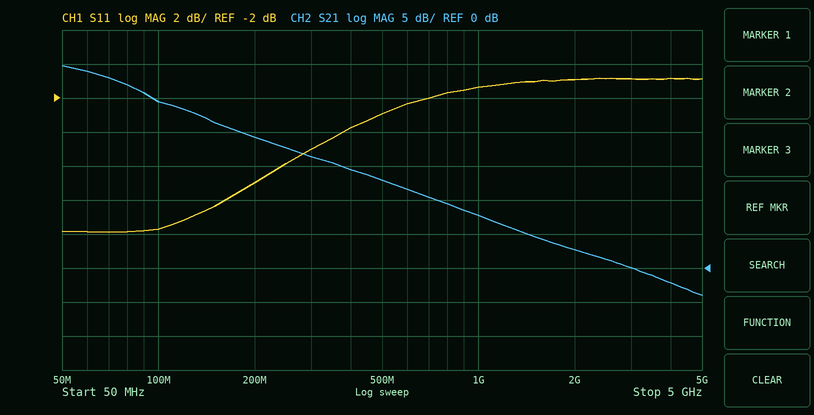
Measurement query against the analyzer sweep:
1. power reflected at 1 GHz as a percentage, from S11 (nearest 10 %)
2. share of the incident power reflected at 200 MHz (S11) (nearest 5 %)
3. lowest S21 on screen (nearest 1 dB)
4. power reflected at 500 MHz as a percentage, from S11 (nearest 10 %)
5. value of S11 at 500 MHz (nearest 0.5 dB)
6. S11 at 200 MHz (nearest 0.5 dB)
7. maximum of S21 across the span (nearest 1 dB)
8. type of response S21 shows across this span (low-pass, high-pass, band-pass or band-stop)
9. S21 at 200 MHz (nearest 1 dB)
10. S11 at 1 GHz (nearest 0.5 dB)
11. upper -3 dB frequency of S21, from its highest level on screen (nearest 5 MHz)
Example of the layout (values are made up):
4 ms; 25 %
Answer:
70 %; 20 %; -4 dB; 50 %; -3.0 dB; -7.0 dB; 30 dB; low-pass; 19 dB; -1.5 dB; 80 MHz
